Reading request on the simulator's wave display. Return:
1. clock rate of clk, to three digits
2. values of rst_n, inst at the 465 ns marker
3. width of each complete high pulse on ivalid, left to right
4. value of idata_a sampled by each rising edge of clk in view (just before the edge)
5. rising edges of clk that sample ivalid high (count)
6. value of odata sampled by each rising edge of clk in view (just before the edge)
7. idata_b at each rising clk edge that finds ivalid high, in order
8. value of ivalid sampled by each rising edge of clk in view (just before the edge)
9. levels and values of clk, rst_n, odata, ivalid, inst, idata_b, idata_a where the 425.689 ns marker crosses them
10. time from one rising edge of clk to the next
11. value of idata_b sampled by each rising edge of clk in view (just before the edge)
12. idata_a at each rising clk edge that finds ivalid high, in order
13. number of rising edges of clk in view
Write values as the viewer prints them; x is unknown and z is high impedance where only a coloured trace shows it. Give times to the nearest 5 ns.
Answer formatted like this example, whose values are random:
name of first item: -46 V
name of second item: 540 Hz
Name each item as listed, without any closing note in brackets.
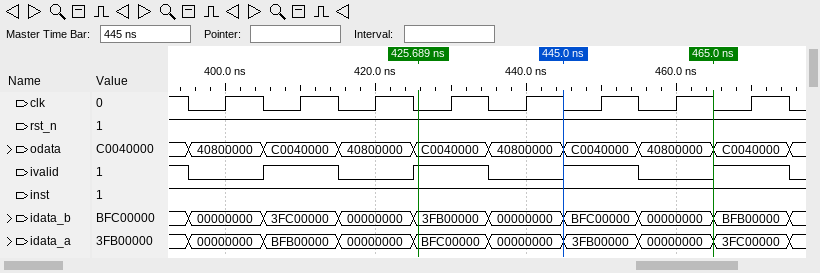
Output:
clock rate of clk, to three digits: 100 MHz
values of rst_n, inst at the 465 ns marker: rst_n=1, inst=1
width of each complete high pulse on ivalid, left to right: 10 ns, 10 ns, 10 ns, 10 ns
value of idata_a sampled by each rising edge of clk in view: 00000000, BFB00000, 00000000, BFC00000, 00000000, 3FB00000, 00000000, 3FC00000
rising edges of clk that sample ivalid high: 4
value of odata sampled by each rising edge of clk in view: 40800000, C0040000, 40800000, C0040000, 40800000, C0040000, 40800000, C0040000
idata_b at each rising clk edge that finds ivalid high, in order: 3FC00000, 3FB00000, BFC00000, BFB00000
value of ivalid sampled by each rising edge of clk in view: 0 1 0 1 0 1 0 1
levels and values of clk, rst_n, odata, ivalid, inst, idata_b, idata_a where the 425.689 ns marker crosses them: clk=0, rst_n=1, odata=C0040000, ivalid=1, inst=1, idata_b=3FB00000, idata_a=BFC00000
time from one rising edge of clk to the next: 10 ns
value of idata_b sampled by each rising edge of clk in view: 00000000, 3FC00000, 00000000, 3FB00000, 00000000, BFC00000, 00000000, BFB00000
idata_a at each rising clk edge that finds ivalid high, in order: BFB00000, BFC00000, 3FB00000, 3FC00000
number of rising edges of clk in view: 8
